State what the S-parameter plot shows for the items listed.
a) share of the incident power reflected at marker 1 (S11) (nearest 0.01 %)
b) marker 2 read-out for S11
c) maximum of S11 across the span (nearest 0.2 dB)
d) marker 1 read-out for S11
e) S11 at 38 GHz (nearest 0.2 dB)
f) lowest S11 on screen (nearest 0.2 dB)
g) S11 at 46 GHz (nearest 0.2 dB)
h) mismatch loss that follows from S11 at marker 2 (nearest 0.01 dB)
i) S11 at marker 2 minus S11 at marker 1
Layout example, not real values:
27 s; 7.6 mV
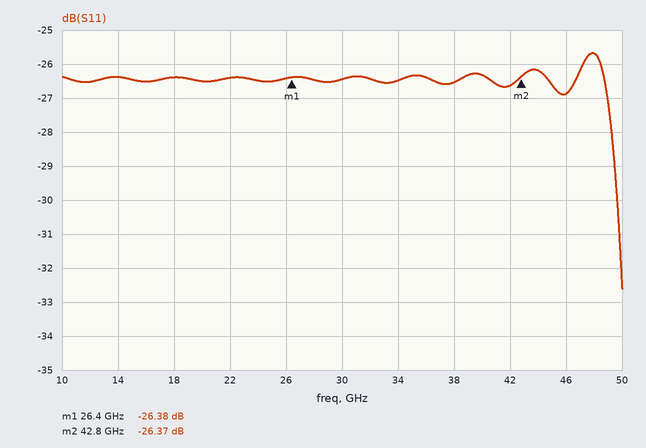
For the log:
0.23 %; -26.37 dB; -25.6 dB; -26.38 dB; -26.6 dB; -32.6 dB; -26.8 dB; 0.01 dB; 0.01 dB
